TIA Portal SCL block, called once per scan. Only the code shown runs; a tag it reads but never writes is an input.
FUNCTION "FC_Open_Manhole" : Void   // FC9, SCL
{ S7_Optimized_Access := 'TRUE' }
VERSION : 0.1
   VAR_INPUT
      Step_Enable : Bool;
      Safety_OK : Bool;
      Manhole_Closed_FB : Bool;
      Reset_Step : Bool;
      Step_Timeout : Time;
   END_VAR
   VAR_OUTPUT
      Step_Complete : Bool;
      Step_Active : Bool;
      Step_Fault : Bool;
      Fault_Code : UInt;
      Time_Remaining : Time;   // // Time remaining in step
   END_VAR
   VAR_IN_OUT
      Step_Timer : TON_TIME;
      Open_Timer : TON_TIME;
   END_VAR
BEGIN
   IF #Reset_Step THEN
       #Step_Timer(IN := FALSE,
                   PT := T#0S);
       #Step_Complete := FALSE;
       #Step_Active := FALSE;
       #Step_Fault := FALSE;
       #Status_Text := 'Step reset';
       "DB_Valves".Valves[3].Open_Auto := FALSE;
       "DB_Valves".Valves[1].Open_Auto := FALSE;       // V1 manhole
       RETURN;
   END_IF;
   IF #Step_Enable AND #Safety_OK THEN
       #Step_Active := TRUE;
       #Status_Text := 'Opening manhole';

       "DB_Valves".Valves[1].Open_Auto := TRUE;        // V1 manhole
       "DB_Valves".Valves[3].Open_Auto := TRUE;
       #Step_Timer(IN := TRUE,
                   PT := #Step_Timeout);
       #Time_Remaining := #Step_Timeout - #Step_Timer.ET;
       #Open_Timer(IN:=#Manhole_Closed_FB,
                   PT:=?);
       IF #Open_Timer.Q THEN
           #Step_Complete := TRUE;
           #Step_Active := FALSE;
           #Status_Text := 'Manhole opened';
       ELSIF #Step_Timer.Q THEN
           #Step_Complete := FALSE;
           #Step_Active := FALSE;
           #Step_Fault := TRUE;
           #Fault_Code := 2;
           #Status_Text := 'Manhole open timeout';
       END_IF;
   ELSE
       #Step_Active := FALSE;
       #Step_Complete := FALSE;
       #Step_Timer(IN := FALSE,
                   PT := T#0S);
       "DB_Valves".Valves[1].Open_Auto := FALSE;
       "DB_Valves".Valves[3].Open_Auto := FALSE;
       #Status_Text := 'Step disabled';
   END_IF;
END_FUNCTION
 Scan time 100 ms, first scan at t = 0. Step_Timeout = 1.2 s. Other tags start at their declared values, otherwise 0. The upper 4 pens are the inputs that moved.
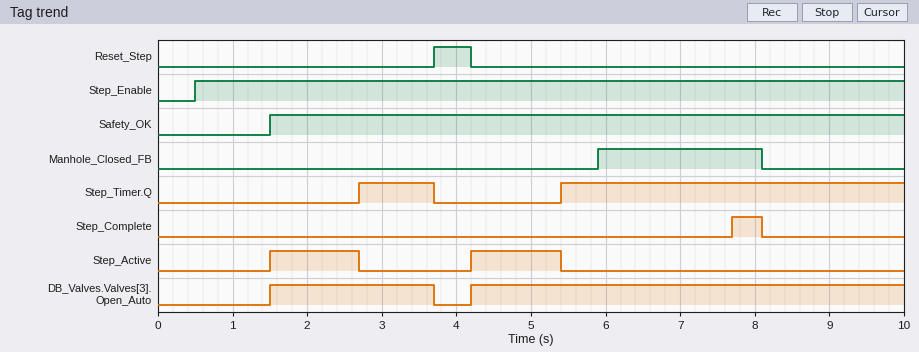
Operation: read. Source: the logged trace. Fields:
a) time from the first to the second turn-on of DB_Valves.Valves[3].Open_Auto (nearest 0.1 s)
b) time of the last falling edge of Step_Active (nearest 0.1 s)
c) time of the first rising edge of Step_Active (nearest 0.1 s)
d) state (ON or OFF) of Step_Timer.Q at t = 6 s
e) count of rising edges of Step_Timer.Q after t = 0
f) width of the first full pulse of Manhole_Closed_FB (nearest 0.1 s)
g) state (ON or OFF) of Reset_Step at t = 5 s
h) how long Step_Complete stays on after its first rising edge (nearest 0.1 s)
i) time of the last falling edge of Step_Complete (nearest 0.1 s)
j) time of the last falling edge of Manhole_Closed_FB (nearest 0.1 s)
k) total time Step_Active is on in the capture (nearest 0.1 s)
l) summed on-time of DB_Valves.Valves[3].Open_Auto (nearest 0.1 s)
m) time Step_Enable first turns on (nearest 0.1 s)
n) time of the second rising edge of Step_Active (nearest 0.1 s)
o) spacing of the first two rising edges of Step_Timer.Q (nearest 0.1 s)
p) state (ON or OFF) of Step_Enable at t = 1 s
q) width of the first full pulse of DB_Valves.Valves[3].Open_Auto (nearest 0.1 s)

2.7 s
5.4 s
1.5 s
ON
2
2.2 s
OFF
0.4 s
8.1 s
8.1 s
2.4 s
8.0 s
0.5 s
4.2 s
2.7 s
ON
2.2 s
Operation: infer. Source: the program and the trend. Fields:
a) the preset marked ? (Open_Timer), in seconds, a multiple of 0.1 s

1.8 s
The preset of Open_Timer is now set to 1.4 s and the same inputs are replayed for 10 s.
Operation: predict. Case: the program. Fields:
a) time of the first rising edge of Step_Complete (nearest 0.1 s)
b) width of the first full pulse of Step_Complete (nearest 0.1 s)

7.3 s
0.8 s
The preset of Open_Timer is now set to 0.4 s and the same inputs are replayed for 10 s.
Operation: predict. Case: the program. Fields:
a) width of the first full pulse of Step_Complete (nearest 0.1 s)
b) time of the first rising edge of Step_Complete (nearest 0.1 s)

1.8 s
6.3 s
